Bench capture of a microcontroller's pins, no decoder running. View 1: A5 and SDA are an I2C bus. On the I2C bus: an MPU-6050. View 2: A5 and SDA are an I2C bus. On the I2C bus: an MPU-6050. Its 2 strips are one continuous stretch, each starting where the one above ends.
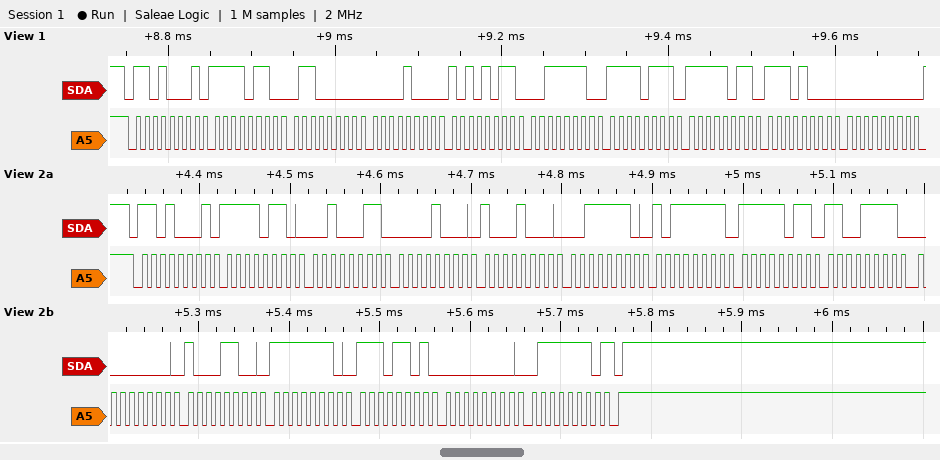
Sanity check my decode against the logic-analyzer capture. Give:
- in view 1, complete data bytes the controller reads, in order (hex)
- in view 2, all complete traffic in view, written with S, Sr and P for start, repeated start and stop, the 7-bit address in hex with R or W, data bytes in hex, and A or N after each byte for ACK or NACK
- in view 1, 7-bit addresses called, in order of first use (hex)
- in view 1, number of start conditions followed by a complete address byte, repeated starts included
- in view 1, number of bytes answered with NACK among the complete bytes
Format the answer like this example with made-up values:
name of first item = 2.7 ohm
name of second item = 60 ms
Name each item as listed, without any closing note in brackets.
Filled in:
in view 1, complete data bytes the controller reads, in order = F6 60 08 AB 3E F7 FB E8 00
in view 2, all complete traffic in view, written with S, Sr and P for start, repeated start and stop, the 7-bit address in hex with R or W, data bytes in hex, and A or N after each byte for ACK or NACK = S 68R A F6 A 23 A 08 A 88 A 3E A BF A FB A CF A 00 A 8C A FE A ED A 00 A 7E N P
in view 1, 7-bit addresses called, in order of first use = 0x68
in view 1, number of start conditions followed by a complete address byte, repeated starts included = 1
in view 1, number of bytes answered with NACK among the complete bytes = 0
